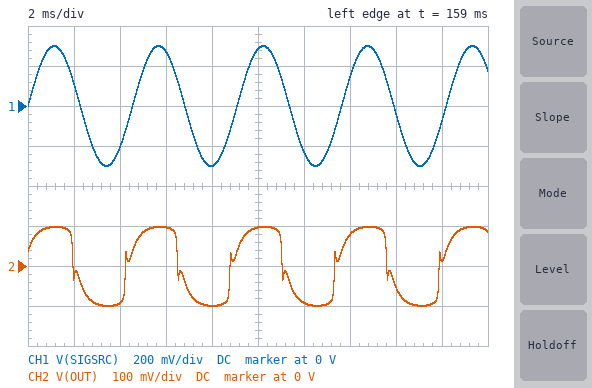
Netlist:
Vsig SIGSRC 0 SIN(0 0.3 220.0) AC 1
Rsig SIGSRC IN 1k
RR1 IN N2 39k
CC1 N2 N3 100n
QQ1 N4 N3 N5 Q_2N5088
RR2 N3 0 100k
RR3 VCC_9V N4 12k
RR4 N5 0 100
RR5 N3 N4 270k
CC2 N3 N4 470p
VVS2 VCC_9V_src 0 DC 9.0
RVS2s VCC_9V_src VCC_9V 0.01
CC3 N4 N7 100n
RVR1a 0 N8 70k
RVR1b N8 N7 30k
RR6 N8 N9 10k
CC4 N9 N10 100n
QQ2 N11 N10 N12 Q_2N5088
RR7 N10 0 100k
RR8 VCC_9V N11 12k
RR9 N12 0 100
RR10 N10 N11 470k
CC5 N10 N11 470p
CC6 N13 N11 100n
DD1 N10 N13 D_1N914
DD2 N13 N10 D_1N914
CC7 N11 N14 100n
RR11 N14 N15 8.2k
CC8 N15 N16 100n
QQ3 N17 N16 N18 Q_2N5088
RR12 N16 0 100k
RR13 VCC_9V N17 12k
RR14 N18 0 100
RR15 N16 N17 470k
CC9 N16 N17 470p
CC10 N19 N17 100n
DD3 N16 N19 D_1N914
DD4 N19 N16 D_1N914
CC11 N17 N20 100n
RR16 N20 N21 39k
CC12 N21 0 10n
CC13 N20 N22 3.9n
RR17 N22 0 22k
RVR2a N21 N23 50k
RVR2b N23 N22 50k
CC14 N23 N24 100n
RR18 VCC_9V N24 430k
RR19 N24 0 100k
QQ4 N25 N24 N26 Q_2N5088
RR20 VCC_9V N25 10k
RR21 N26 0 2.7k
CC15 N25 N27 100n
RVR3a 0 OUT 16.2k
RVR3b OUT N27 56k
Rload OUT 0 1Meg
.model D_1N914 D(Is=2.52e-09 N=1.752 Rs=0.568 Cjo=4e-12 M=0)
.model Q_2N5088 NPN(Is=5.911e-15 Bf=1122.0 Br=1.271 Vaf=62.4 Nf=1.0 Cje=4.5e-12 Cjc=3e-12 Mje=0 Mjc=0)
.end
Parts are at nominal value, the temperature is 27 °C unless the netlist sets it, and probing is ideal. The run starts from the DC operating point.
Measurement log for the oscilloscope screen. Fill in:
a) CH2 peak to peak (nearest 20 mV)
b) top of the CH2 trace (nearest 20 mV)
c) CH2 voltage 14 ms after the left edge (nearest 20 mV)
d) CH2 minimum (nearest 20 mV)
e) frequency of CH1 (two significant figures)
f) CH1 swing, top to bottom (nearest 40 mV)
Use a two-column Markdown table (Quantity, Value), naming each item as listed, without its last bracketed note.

| Quantity | Value |
|---|---|
| CH2 peak to peak | 200 mV |
| top of the CH2 trace | 100 mV |
| CH2 voltage 14 ms after the left edge | 80 mV |
| CH2 minimum | -100 mV |
| frequency of CH1 | 220 Hz |
| CH1 swing, top to bottom | 600 mV |
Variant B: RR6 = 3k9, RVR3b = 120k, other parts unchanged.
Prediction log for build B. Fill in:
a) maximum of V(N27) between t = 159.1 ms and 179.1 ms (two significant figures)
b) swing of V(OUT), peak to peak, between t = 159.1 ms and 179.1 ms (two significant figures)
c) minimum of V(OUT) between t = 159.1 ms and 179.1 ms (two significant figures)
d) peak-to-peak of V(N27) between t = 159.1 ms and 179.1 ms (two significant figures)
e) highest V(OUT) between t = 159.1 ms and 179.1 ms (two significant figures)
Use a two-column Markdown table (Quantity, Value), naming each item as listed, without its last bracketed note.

| Quantity | Value |
|---|---|
| maximum of V(N27) between t = 159.1 ms and 179.1 ms | 490 mV |
| swing of V(OUT), peak to peak, between t = 159.1 ms and 179.1 ms | 120 mV |
| minimum of V(OUT) between t = 159.1 ms and 179.1 ms | -59 mV |
| peak-to-peak of V(N27) between t = 159.1 ms and 179.1 ms | 990 mV |
| highest V(OUT) between t = 159.1 ms and 179.1 ms | 57 mV |
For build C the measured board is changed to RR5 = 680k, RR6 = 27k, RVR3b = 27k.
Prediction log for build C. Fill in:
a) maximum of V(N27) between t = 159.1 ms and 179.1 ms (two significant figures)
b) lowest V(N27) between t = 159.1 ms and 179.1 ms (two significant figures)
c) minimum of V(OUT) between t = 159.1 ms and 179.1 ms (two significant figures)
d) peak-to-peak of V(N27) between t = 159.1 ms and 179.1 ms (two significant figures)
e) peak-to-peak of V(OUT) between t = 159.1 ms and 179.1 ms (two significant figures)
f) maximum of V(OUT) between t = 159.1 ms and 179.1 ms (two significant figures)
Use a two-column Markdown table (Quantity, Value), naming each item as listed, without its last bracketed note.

| Quantity | Value |
|---|---|
| maximum of V(N27) between t = 159.1 ms and 179.1 ms | 420 mV |
| lowest V(N27) between t = 159.1 ms and 179.1 ms | -410 mV |
| minimum of V(OUT) between t = 159.1 ms and 179.1 ms | -150 mV |
| peak-to-peak of V(N27) between t = 159.1 ms and 179.1 ms | 830 mV |
| peak-to-peak of V(OUT) between t = 159.1 ms and 179.1 ms | 310 mV |
| maximum of V(OUT) between t = 159.1 ms and 179.1 ms | 160 mV |
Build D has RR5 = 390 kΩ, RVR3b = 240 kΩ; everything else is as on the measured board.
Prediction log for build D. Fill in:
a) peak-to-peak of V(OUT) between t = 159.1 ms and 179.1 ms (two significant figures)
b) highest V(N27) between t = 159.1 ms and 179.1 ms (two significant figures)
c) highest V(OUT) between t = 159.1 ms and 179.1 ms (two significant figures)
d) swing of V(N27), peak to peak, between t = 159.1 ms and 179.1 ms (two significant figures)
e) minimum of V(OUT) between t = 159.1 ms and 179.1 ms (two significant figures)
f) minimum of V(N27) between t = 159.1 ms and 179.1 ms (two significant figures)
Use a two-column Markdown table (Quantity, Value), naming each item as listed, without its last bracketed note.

| Quantity | Value |
|---|---|
| peak-to-peak of V(OUT) between t = 159.1 ms and 179.1 ms | 66 mV |
| highest V(N27) between t = 159.1 ms and 179.1 ms | 520 mV |
| highest V(OUT) between t = 159.1 ms and 179.1 ms | 32 mV |
| swing of V(N27), peak to peak, between t = 159.1 ms and 179.1 ms | 1.1 V |
| minimum of V(OUT) between t = 159.1 ms and 179.1 ms | -34 mV |
| minimum of V(N27) between t = 159.1 ms and 179.1 ms | -540 mV |
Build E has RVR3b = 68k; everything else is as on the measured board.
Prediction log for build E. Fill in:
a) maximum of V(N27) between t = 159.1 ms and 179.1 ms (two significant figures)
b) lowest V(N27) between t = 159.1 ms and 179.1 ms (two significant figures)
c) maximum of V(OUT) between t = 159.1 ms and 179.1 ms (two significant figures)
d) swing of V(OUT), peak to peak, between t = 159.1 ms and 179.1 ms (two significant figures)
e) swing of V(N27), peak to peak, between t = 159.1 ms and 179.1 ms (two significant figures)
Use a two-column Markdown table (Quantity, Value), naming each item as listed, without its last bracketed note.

| Quantity | Value |
|---|---|
| maximum of V(N27) between t = 159.1 ms and 179.1 ms | 450 mV |
| lowest V(N27) between t = 159.1 ms and 179.1 ms | -460 mV |
| maximum of V(OUT) between t = 159.1 ms and 179.1 ms | 86 mV |
| swing of V(OUT), peak to peak, between t = 159.1 ms and 179.1 ms | 170 mV |
| swing of V(N27), peak to peak, between t = 159.1 ms and 179.1 ms | 910 mV |
